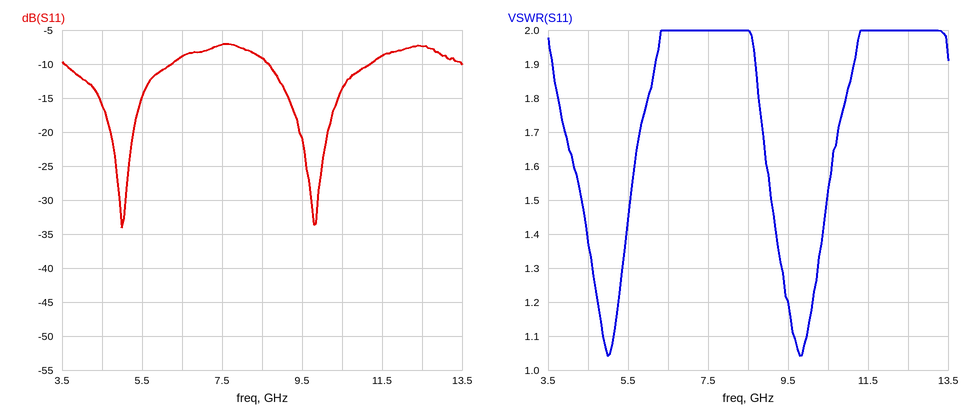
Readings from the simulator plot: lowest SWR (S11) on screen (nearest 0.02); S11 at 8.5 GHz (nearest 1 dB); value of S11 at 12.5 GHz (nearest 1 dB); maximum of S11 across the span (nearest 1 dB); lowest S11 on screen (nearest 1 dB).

1.04
-9 dB
-7 dB
-7 dB
-34 dB
